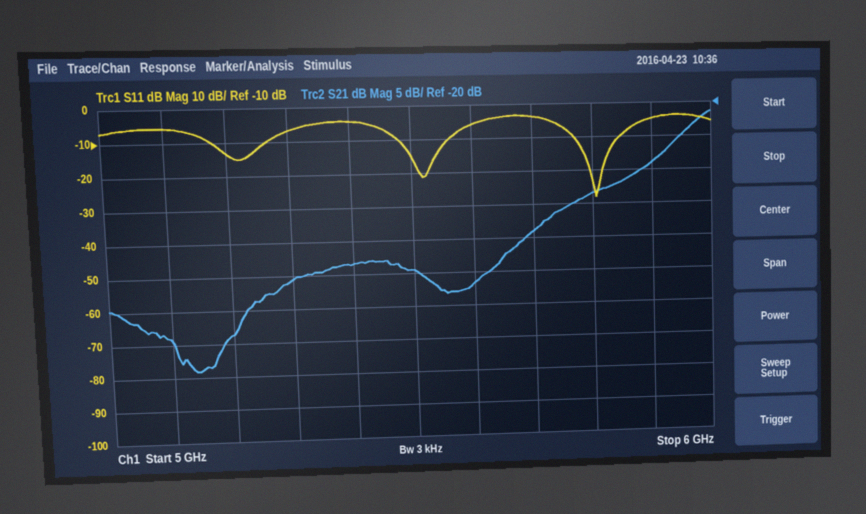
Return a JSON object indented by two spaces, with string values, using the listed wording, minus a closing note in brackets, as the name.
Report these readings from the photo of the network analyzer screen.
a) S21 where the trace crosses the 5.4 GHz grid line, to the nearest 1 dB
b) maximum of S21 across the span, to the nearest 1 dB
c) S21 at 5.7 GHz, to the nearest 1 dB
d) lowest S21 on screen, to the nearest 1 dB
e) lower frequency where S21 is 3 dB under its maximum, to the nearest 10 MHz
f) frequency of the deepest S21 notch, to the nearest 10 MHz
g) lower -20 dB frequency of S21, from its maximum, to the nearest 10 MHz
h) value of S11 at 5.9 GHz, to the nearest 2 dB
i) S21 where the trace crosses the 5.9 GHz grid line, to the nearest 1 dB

{
  "S21 where the trace crosses the 5.4 GHz grid line, to the nearest 1 dB": "-43 dB",
  "maximum of S21 across the span, to the nearest 1 dB": "-21 dB",
  "S21 at 5.7 GHz, to the nearest 1 dB": "-39 dB",
  "lowest S21 on screen, to the nearest 1 dB": "-59 dB",
  "lower frequency where S21 is 3 dB under its maximum, to the nearest 10 MHz": "5.96 GHz",
  "frequency of the deepest S21 notch, to the nearest 10 MHz": "5.14 GHz",
  "lower -20 dB frequency of S21, from its maximum, to the nearest 10 MHz": "5.67 GHz",
  "value of S11 at 5.9 GHz, to the nearest 2 dB": "-4 dB",
  "S21 where the trace crosses the 5.9 GHz grid line, to the nearest 1 dB": "-29 dB"
}
